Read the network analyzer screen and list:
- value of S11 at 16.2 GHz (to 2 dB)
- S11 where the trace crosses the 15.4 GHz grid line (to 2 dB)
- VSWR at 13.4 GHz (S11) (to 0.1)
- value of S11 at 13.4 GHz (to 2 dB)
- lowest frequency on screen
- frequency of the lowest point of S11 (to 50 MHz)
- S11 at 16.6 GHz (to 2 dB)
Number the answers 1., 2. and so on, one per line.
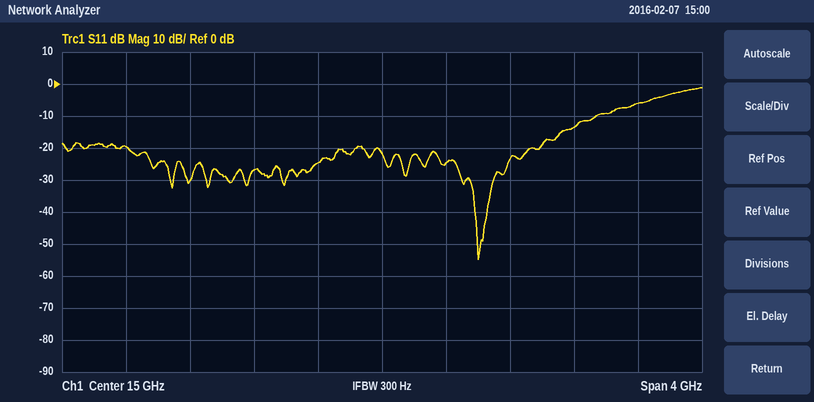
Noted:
1. -14 dB
2. -24 dB
3. 1.2
4. -20 dB
5. 13 GHz
6. 15.60 GHz
7. -6 dB
